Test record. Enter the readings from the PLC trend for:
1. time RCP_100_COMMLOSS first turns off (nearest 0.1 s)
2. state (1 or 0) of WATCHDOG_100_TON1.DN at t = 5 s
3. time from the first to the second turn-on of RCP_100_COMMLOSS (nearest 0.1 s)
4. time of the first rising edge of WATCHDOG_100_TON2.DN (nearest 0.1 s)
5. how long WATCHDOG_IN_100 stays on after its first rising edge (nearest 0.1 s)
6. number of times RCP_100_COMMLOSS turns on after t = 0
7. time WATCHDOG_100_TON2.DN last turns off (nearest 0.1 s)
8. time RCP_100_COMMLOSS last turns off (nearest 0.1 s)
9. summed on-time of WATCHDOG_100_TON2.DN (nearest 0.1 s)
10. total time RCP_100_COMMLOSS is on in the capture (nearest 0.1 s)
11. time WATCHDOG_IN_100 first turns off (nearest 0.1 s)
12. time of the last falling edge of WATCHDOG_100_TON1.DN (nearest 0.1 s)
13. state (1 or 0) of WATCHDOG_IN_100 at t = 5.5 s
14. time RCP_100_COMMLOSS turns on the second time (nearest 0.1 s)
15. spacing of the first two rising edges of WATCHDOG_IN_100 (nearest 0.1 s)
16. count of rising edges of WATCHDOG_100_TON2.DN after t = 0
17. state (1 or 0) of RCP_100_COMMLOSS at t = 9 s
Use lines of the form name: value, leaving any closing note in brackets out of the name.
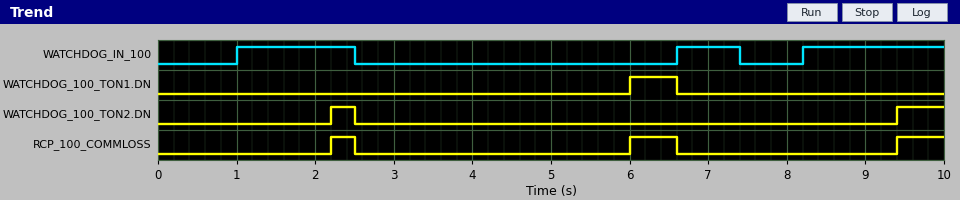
time RCP_100_COMMLOSS first turns off: 2.5 s
state (1 or 0) of WATCHDOG_100_TON1.DN at t = 5 s: 0
time from the first to the second turn-on of RCP_100_COMMLOSS: 3.8 s
time of the first rising edge of WATCHDOG_100_TON2.DN: 2.2 s
how long WATCHDOG_IN_100 stays on after its first rising edge: 1.5 s
number of times RCP_100_COMMLOSS turns on after t = 0: 3
time WATCHDOG_100_TON2.DN last turns off: 2.5 s
time RCP_100_COMMLOSS last turns off: 6.6 s
summed on-time of WATCHDOG_100_TON2.DN: 0.9 s
total time RCP_100_COMMLOSS is on in the capture: 1.5 s
time WATCHDOG_IN_100 first turns off: 2.5 s
time of the last falling edge of WATCHDOG_100_TON1.DN: 6.6 s
state (1 or 0) of WATCHDOG_IN_100 at t = 5.5 s: 0
time RCP_100_COMMLOSS turns on the second time: 6.0 s
spacing of the first two rising edges of WATCHDOG_IN_100: 5.6 s
count of rising edges of WATCHDOG_100_TON2.DN after t = 0: 2
state (1 or 0) of RCP_100_COMMLOSS at t = 9 s: 0
